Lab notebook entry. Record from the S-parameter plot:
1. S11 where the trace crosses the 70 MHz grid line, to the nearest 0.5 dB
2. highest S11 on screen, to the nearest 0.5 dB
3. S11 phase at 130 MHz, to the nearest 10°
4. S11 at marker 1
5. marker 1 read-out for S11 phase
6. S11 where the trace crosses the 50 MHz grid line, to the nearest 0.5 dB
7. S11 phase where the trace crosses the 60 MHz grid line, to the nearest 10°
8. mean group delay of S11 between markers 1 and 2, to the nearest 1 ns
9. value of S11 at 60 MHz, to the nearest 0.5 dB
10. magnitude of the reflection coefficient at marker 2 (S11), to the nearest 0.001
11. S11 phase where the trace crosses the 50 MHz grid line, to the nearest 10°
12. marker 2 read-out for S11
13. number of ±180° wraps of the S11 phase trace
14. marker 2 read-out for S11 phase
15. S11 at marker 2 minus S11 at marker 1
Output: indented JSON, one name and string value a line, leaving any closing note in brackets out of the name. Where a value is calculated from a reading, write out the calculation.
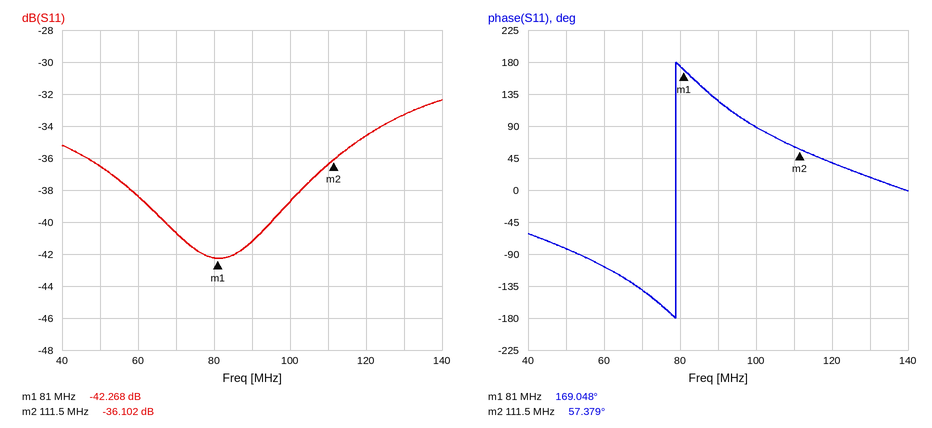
{
  "S11 where the trace crosses the 70 MHz grid line, to the nearest 0.5 dB": "-40.5 dB",
  "highest S11 on screen, to the nearest 0.5 dB": "-32.5 dB",
  "S11 phase at 130 MHz, to the nearest 10°": "20°",
  "S11 at marker 1": "-42.268 dB",
  "marker 1 read-out for S11 phase": "169.048°",
  "S11 where the trace crosses the 50 MHz grid line, to the nearest 0.5 dB": "-36.5 dB",
  "S11 phase where the trace crosses the 60 MHz grid line, to the nearest 10°": "-110°",
  "mean group delay of S11 between markers 1 and 2, to the nearest 1 ns": "−(57.379° − (169.048°))/(360° × 30.5 MHz) ≈ 10 ns",
  "value of S11 at 60 MHz, to the nearest 0.5 dB": "-38.5 dB",
  "magnitude of the reflection coefficient at marker 2 (S11), to the nearest 0.001": "10^(-36.102/20) ≈ 0.016",
  "S11 phase where the trace crosses the 50 MHz grid line, to the nearest 10°": "-80°",
  "marker 2 read-out for S11": "-36.102 dB",
  "number of ±180° wraps of the S11 phase trace": "1",
  "marker 2 read-out for S11 phase": "57.379°",
  "S11 at marker 2 minus S11 at marker 1": "-36.102 − (-42.268) = 6.166 dB"
}
